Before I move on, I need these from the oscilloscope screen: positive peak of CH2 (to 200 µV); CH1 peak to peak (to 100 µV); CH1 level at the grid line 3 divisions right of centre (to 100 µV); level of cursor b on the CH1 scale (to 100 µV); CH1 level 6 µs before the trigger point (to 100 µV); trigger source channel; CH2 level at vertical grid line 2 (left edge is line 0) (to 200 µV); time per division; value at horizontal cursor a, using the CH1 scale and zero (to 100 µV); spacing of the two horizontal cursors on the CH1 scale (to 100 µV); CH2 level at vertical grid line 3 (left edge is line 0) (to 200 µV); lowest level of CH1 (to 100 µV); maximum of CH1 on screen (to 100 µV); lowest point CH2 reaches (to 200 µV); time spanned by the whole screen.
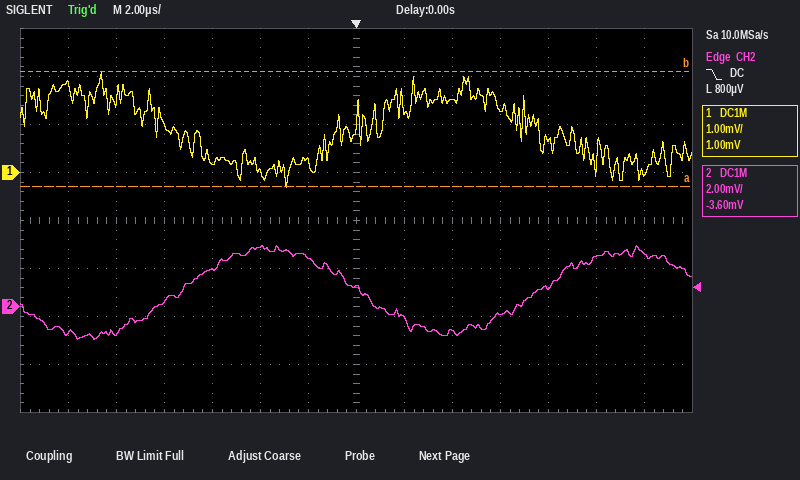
2.6 mV
2.4 mV
1.3 mV
2.1 mV
200 µV
CH2
-1.2 mV
2 µs
-300 µV
2.4 mV
200 µV
-300 µV
2.1 mV
-1.4 mV
28 µs
